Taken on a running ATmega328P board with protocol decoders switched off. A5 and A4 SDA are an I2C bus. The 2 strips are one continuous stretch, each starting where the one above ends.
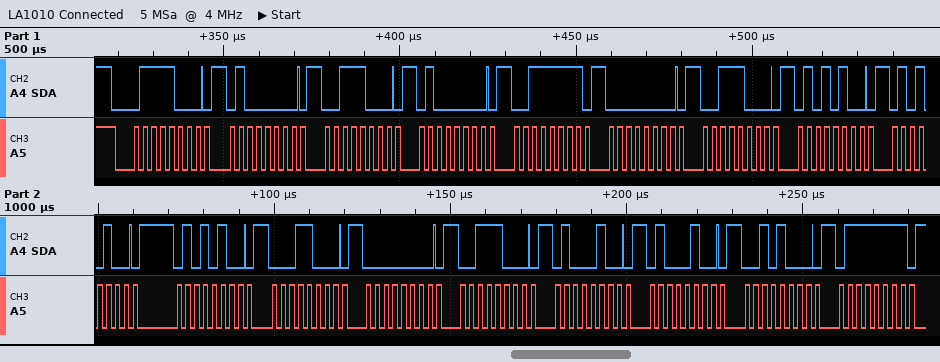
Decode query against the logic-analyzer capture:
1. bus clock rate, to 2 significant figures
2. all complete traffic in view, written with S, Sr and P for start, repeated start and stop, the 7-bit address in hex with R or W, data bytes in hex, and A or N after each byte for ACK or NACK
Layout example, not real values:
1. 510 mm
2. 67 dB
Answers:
1. 400 kHz
2. S 3CW A 40 A 38 A 40 A 3F A 00 A 38 A 54 A 54 A 54 A 18 A 00 A 38 A 44 A 44 A 28 A 7F A
